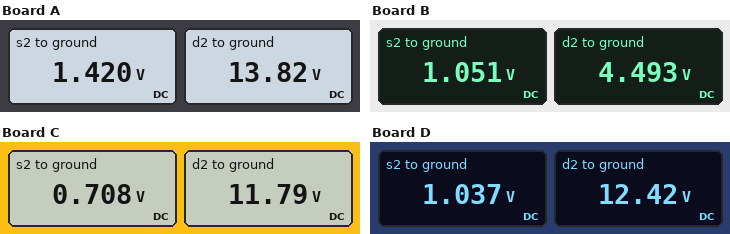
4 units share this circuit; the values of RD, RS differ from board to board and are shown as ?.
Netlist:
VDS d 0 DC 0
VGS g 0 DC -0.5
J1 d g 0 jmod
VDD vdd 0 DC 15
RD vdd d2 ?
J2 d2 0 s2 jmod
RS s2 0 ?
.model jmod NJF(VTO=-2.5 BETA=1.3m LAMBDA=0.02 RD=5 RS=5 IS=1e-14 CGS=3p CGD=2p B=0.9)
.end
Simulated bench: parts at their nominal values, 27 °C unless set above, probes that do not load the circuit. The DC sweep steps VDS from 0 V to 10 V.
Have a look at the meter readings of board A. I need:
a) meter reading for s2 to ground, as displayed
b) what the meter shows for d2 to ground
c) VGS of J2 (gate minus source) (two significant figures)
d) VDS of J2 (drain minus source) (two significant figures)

1.420 V
13.82 V
-1.4 V
12 V
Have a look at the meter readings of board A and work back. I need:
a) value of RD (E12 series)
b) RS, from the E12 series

680 Ω
820 Ω
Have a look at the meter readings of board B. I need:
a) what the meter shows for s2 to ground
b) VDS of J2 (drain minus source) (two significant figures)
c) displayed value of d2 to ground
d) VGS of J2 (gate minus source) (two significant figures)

1.051 V
3.4 V
4.493 V
-1.1 V
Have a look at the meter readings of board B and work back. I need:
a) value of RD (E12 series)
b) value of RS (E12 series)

3.9 kΩ
390 Ω
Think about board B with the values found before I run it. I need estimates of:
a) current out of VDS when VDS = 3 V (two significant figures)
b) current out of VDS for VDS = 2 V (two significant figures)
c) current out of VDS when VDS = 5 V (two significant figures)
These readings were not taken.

5.1 mA
5.0 mA
5.3 mA
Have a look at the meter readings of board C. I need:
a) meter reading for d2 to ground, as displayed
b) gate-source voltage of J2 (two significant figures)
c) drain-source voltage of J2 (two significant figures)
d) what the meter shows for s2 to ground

11.79 V
-710 mV
11 V
0.708 V
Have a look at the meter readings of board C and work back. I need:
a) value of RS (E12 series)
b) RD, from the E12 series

150 Ω
680 Ω
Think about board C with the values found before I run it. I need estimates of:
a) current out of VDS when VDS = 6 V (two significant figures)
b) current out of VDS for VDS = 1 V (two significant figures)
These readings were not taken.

5.4 mA
3.7 mA
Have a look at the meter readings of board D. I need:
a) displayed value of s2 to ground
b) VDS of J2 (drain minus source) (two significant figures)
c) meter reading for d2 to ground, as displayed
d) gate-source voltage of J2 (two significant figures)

1.037 V
11 V
12.42 V
-1.0 V
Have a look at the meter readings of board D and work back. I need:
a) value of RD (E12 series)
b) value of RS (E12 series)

820 Ω
330 Ω
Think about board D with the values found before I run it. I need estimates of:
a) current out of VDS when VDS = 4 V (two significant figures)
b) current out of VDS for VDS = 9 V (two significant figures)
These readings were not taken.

5.2 mA
5.7 mA
